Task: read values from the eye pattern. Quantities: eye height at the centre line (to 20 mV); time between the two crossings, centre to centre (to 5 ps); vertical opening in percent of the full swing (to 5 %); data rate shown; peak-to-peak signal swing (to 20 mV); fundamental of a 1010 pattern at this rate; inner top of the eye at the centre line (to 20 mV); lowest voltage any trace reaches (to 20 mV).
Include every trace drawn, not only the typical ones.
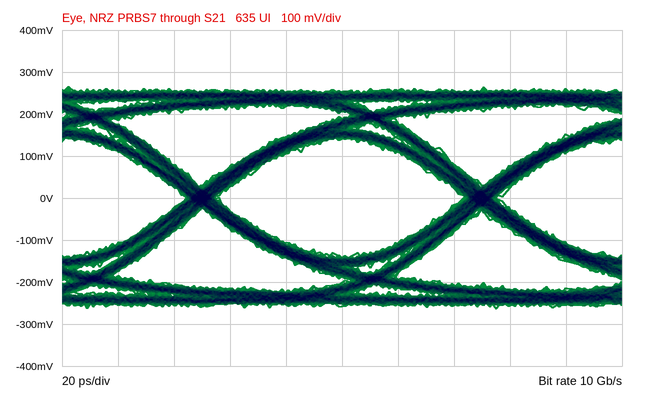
280 mV
100 ps
55 %
10 Gb/s
520 mV
5 GHz
140 mV
-260 mV
